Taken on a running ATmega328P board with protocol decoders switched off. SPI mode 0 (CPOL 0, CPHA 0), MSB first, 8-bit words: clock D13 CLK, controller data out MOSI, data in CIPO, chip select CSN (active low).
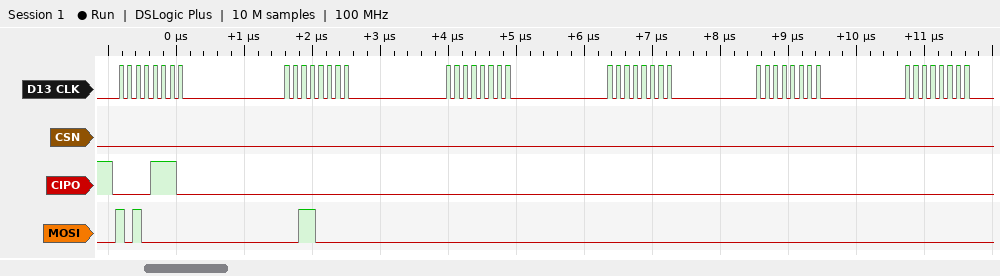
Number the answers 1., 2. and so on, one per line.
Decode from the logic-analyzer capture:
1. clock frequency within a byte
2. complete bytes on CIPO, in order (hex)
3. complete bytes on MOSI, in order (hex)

1. 8 MHz
2. 0E 00 00 00 00 00
3. A0 30 00 00 00 00
